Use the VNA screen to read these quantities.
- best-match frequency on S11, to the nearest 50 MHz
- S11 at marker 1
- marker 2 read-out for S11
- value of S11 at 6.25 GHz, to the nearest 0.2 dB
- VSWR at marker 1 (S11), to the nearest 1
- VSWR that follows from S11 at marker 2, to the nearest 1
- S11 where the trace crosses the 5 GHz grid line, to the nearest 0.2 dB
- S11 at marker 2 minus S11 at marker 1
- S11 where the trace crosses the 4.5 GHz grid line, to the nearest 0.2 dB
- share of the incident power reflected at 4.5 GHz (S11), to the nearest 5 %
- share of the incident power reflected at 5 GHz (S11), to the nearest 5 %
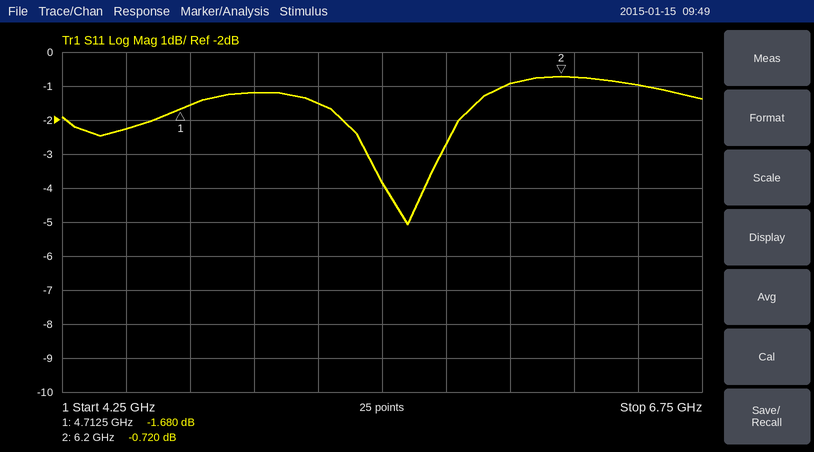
5.60 GHz
-1.680 dB
-0.720 dB
-0.8 dB
10
24
-1.2 dB
0.960 dB
-2.2 dB
60 %
75 %
